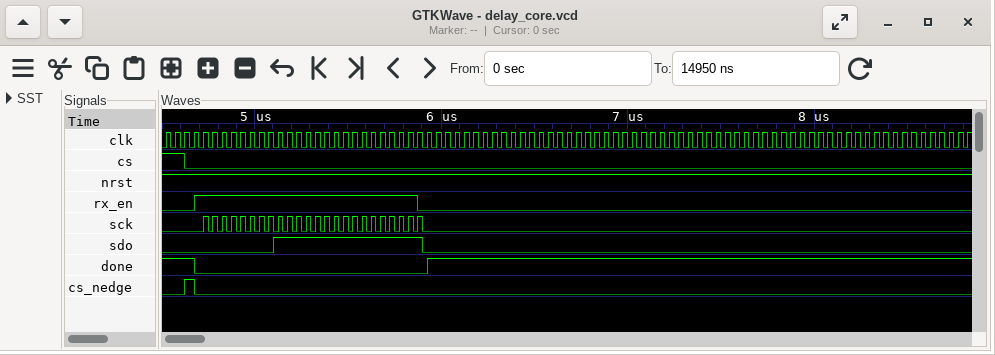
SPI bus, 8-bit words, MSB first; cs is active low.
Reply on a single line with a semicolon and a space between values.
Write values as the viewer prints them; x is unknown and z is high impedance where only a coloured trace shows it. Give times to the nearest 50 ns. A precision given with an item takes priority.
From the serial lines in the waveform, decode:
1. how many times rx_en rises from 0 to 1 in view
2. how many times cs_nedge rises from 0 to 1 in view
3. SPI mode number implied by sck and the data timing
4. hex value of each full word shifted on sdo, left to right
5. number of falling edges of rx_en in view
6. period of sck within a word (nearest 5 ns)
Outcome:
1; 1; 0; 00, FF, FF; 1; 50 ns
